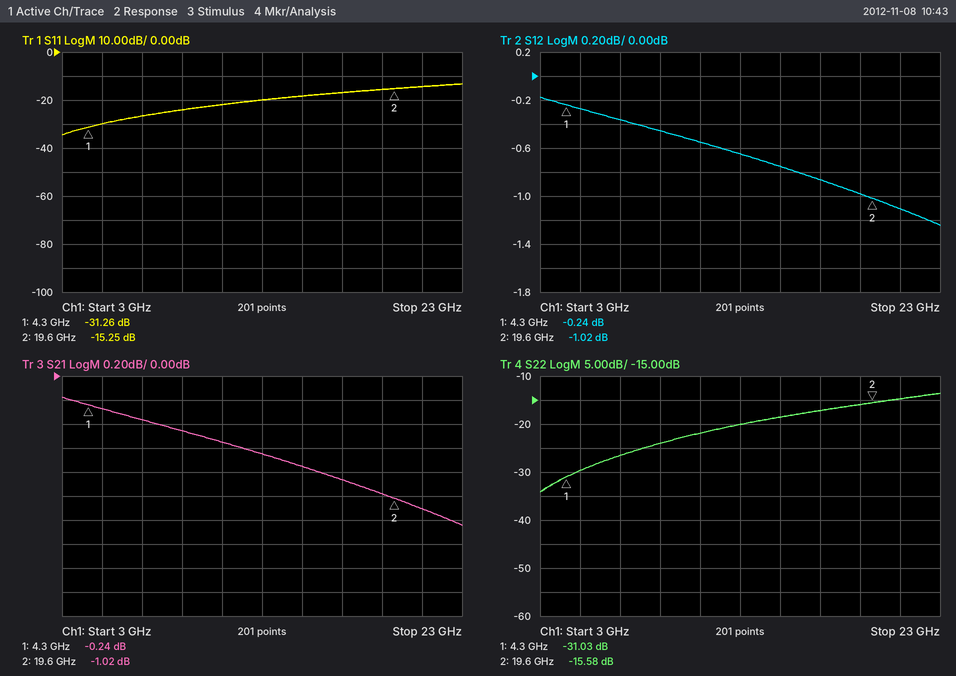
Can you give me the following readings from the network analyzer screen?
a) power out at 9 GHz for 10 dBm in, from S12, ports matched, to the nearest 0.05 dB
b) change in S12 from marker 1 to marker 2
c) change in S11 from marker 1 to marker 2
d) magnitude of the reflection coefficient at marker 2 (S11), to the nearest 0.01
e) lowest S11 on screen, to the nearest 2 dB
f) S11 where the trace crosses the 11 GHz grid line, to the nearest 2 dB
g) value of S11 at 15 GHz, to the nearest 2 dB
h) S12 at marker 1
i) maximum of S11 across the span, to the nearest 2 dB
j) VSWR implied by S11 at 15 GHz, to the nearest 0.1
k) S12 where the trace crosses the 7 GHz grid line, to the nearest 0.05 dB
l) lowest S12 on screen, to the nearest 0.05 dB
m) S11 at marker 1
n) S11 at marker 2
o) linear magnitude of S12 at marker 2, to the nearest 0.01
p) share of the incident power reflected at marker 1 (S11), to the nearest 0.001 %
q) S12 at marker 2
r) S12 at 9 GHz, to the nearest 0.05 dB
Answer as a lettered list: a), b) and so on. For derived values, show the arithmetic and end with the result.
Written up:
a) 10 dBm + (-0.45 dB) = 9.55 dBm
b) -1.02 − (-0.24) = -0.78 dB
c) -15.25 − (-31.26) = 16.01 dB
d) 10^(-15.25/20) ≈ 0.17
e) -34 dB
f) -22 dB
g) -18 dB
h) -0.24 dB
i) -14 dB
j) |Γ| = 10^(-18/20) = 0.1259; VSWR = (1 + 0.1259)/(1 − 0.1259) ≈ 1.3
k) -0.35 dB
l) -1.25 dB
m) -31.26 dB
n) -15.25 dB
o) 10^(-1.02/20) ≈ 0.89
p) 10^(-31.26/10) ≈ 0.075 %
q) -1.02 dB
r) -0.45 dB
